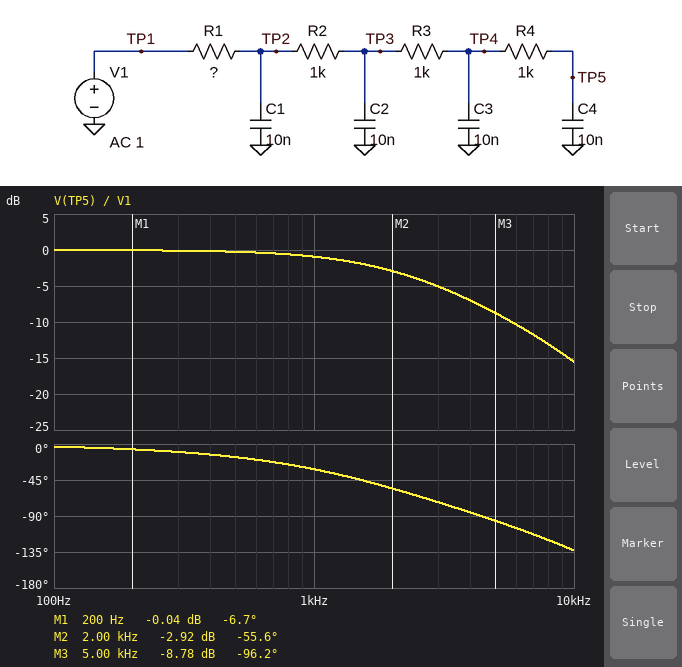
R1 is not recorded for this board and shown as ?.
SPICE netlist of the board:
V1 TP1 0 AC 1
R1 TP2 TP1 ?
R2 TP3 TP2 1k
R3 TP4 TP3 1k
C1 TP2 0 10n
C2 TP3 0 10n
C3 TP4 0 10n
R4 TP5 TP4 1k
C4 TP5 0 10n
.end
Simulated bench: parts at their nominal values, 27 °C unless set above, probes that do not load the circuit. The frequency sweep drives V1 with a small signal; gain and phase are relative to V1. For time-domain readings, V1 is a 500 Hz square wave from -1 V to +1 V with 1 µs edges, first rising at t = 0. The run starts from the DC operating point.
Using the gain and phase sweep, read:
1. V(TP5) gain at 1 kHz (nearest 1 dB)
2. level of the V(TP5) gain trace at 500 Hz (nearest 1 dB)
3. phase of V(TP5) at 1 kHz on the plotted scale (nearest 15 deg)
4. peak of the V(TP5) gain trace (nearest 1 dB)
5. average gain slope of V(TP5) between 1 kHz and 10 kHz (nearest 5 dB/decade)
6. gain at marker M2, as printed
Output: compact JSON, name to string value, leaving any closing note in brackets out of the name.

{"V(TP5) gain at 1 kHz": "-1 dB", "level of the V(TP5) gain trace at 500 Hz": "0 dB", "phase of V(TP5) at 1 kHz on the plotted scale": "-30 deg", "peak of the V(TP5) gain trace": "0 dB", "average gain slope of V(TP5) between 1 kHz and 10 kHz": "-15 dB/decade", "gain at marker M2, as printed": "-2.92 dB"}
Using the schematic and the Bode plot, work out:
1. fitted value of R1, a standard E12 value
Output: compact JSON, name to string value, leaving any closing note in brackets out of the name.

{"fitted value of R1, a standard E12 value": "820 Ω"}
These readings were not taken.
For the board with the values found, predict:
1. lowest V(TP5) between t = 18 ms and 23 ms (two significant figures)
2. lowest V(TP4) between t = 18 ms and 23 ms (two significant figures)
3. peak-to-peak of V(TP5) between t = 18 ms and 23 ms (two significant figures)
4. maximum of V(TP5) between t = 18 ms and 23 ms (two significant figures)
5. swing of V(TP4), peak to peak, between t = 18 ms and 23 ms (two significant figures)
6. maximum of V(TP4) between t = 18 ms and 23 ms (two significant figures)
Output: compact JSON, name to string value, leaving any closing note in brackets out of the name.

{"lowest V(TP5) between t = 18 ms and 23 ms": "-1.0 V", "lowest V(TP4) between t = 18 ms and 23 ms": "-1.0 V", "peak-to-peak of V(TP5) between t = 18 ms and 23 ms": "2.0 V", "maximum of V(TP5) between t = 18 ms and 23 ms": "1.0 V", "swing of V(TP4), peak to peak, between t = 18 ms and 23 ms": "2.0 V", "maximum of V(TP4) between t = 18 ms and 23 ms": "1.0 V"}
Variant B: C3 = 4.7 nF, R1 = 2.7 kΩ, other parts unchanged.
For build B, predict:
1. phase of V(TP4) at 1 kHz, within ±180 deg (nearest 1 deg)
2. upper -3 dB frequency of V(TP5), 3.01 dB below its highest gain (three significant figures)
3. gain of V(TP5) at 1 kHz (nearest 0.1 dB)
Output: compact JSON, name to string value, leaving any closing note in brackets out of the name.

{"phase of V(TP4) at 1 kHz, within ±180 deg": "-41 deg", "upper -3 dB frequency of V(TP5), 3.01 dB below its highest gain": "1.27 kHz", "gain of V(TP5) at 1 kHz": "-2.1 dB"}
